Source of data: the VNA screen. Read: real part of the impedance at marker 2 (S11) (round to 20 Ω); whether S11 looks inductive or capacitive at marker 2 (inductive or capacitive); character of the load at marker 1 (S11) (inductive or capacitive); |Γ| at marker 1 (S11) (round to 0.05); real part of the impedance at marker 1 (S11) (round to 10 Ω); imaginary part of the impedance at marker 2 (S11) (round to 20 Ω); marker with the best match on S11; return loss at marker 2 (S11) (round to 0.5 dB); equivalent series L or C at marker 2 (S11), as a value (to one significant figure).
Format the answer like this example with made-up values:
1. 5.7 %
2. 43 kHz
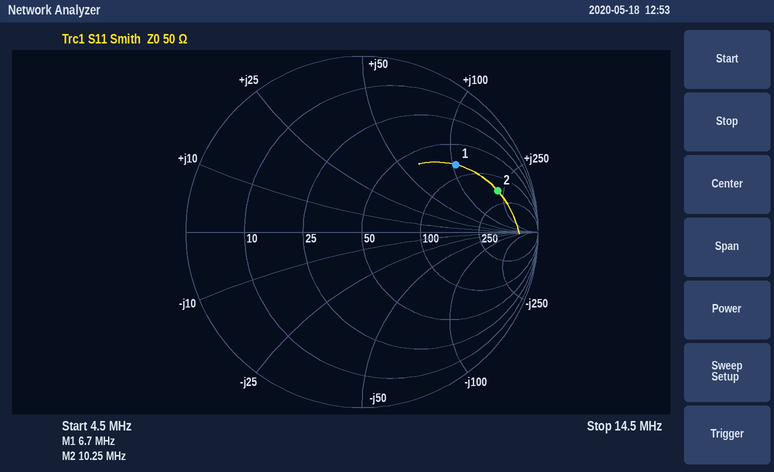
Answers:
1. 160 Ω
2. inductive
3. inductive
4. 0.65
5. 80 Ω
6. +220 Ω
7. marker 1
8. 2.0 dB
9. 3 µH
